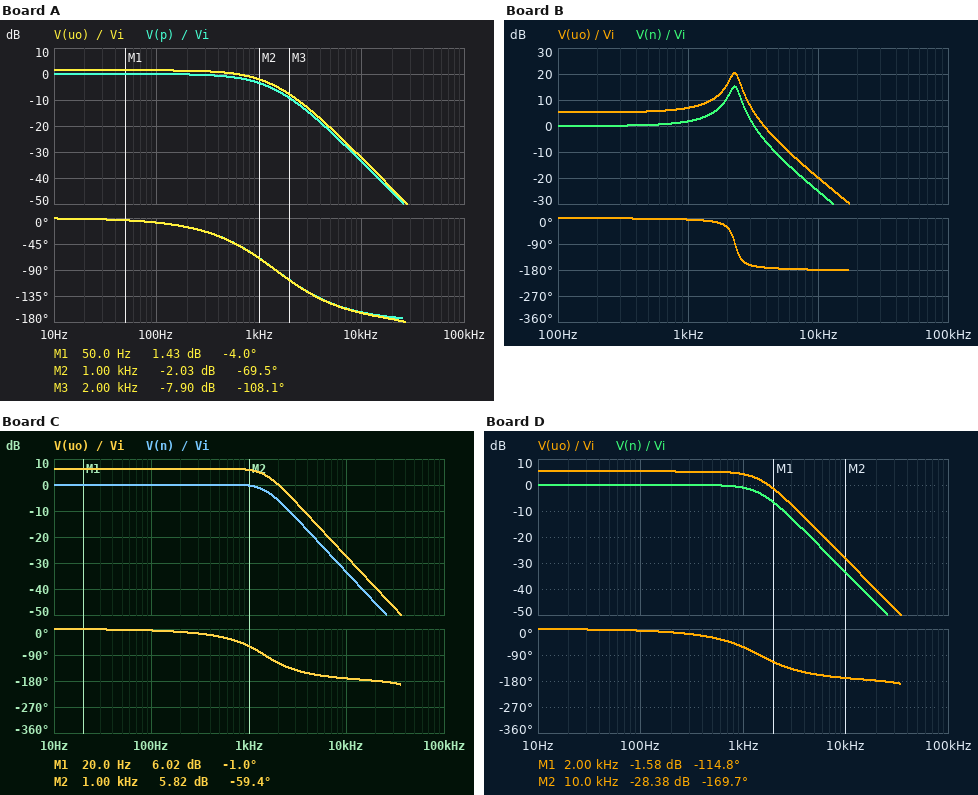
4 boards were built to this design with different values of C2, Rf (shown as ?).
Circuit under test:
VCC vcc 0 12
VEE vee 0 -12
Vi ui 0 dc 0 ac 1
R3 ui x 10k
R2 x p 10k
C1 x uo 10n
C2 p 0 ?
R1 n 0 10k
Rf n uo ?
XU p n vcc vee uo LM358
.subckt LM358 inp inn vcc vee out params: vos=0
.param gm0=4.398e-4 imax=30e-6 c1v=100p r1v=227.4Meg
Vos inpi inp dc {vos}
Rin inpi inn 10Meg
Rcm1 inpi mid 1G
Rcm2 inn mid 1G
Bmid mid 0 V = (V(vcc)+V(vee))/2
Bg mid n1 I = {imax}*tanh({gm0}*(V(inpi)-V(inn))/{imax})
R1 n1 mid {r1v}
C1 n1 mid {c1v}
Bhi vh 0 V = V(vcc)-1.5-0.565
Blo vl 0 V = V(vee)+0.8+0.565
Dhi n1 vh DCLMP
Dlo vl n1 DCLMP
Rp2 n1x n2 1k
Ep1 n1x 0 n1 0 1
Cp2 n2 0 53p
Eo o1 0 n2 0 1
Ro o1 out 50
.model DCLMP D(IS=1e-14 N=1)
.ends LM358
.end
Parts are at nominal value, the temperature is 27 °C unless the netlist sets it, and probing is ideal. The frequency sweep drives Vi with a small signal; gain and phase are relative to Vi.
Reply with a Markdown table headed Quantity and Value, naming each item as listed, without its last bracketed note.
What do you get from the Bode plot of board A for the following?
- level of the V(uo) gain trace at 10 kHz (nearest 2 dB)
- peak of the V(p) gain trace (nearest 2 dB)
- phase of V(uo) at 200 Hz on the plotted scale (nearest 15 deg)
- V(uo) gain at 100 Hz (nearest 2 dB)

| Quantity | Value |
|---|---|
| level of the V(uo) gain trace at 10 kHz | -32 dB |
| peak of the V(p) gain trace | 0 dB |
| phase of V(uo) at 200 Hz on the plotted scale | -15 deg |
| V(uo) gain at 100 Hz | 2 dB |
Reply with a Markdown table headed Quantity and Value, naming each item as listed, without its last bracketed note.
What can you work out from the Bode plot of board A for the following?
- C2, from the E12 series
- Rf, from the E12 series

| Quantity | Value |
|---|---|
| C2, from the E12 series | 12 nF |
| Rf, from the E12 series | 1.8 kΩ |
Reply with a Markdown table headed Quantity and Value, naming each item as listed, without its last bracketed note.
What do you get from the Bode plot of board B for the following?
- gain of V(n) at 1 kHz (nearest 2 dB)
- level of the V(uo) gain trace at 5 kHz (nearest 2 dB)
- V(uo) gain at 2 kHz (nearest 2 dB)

| Quantity | Value |
|---|---|
| gain of V(n) at 1 kHz | 2 dB |
| level of the V(uo) gain trace at 5 kHz | -6 dB |
| V(uo) gain at 2 kHz | 16 dB |
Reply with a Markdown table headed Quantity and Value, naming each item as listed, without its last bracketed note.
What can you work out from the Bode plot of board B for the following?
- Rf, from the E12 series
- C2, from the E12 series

| Quantity | Value |
|---|---|
| Rf, from the E12 series | 8.2 kΩ |
| C2, from the E12 series | 4.7 nF |
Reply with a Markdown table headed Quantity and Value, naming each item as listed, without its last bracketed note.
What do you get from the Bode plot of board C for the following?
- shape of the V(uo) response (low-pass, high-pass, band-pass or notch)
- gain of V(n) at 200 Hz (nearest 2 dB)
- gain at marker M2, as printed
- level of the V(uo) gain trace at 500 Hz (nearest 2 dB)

| Quantity | Value |
|---|---|
| shape of the V(uo) response | low-pass |
| gain of V(n) at 200 Hz | 0 dB |
| gain at marker M2, as printed | 5.82 dB |
| level of the V(uo) gain trace at 500 Hz | 6 dB |
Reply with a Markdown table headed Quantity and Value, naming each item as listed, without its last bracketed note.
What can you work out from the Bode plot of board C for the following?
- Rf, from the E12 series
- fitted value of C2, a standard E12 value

| Quantity | Value |
|---|---|
| Rf, from the E12 series | 10 kΩ |
| fitted value of C2, a standard E12 value | 12 nF |
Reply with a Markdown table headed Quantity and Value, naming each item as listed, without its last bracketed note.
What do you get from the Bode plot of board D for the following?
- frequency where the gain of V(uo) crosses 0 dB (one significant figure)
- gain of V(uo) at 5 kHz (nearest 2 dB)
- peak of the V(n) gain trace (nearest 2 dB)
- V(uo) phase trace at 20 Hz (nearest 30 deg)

| Quantity | Value |
|---|---|
| frequency where the gain of V(uo) crosses 0 dB | 2 kHz |
| gain of V(uo) at 5 kHz | -16 dB |
| peak of the V(n) gain trace | 0 dB |
| V(uo) phase trace at 20 Hz | 0 deg |
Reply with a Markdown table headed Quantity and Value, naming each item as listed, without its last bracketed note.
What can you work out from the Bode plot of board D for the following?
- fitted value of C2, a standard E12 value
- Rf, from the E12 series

| Quantity | Value |
|---|---|
| fitted value of C2, a standard E12 value | 12 nF |
| Rf, from the E12 series | 8.2 kΩ |
